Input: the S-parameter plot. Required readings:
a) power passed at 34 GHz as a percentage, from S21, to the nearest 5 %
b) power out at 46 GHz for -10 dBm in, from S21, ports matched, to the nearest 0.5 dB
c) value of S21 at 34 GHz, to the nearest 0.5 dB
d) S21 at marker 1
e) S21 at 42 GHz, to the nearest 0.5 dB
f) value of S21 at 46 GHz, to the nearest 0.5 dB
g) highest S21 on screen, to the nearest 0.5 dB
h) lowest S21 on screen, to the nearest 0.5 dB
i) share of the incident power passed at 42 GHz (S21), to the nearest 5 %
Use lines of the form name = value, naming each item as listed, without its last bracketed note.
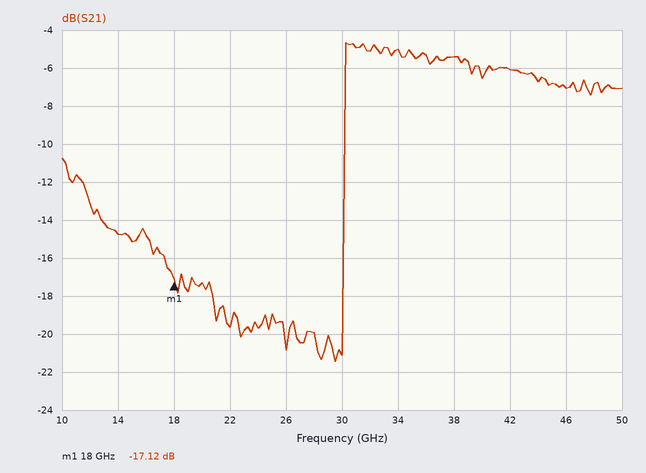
power passed at 34 GHz as a percentage, from S21, to the nearest 5 % = 30 %
power out at 46 GHz for -10 dBm in, from S21, ports matched, to the nearest 0.5 dB = -17.0 dBm
value of S21 at 34 GHz, to the nearest 0.5 dB = -5.0 dB
S21 at marker 1 = -17.12 dB
S21 at 42 GHz, to the nearest 0.5 dB = -6.0 dB
value of S21 at 46 GHz, to the nearest 0.5 dB = -7.0 dB
highest S21 on screen, to the nearest 0.5 dB = -4.5 dB
lowest S21 on screen, to the nearest 0.5 dB = -21.5 dB
share of the incident power passed at 42 GHz (S21), to the nearest 5 % = 25 %
